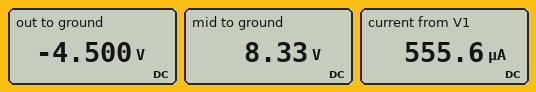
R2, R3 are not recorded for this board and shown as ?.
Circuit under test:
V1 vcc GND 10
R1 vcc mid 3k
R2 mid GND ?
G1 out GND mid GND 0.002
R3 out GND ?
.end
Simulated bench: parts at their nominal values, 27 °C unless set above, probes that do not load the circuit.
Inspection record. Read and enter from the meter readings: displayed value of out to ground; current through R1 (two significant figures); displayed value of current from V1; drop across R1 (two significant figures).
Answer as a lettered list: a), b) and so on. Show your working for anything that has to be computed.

a) -4.500 V
b) (10 V - 8.33 V) / 3 kΩ = 560 µA
c) 555.6 µA
d) 10 V - 8.33 V = 1.7 V
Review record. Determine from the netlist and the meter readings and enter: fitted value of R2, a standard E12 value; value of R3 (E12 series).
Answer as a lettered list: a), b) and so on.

a) 15 kΩ
b) 270 Ω
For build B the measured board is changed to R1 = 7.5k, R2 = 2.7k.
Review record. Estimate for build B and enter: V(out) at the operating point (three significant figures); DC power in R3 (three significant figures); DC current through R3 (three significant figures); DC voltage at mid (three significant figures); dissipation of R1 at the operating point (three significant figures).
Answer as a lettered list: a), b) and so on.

a) -1.43 V
b) 7.57 mW
c) 5.29 mA
d) 2.65 V
e) 7.21 mW
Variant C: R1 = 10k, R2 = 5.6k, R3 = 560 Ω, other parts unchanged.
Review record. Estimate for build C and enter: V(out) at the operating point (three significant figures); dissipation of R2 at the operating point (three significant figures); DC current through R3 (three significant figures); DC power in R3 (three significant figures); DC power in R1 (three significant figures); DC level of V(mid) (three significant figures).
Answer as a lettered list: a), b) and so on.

a) -4.02 V
b) 2.30 mW
c) 7.18 mA
d) 28.9 mW
e) 4.11 mW
f) 3.59 V
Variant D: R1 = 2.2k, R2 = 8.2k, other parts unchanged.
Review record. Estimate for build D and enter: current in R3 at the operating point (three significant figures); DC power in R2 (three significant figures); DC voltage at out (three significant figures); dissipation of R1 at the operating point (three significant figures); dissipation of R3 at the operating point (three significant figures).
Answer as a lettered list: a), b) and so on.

a) 15.8 mA
b) 7.58 mW
c) -4.26 V
d) 2.03 mW
e) 67.1 mW
